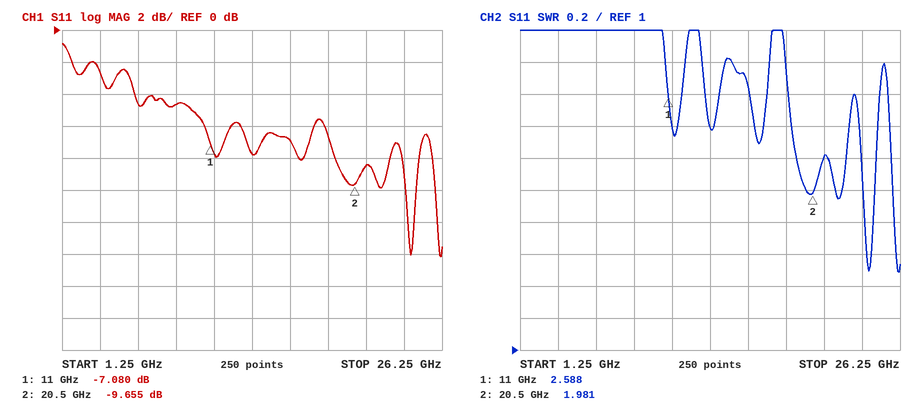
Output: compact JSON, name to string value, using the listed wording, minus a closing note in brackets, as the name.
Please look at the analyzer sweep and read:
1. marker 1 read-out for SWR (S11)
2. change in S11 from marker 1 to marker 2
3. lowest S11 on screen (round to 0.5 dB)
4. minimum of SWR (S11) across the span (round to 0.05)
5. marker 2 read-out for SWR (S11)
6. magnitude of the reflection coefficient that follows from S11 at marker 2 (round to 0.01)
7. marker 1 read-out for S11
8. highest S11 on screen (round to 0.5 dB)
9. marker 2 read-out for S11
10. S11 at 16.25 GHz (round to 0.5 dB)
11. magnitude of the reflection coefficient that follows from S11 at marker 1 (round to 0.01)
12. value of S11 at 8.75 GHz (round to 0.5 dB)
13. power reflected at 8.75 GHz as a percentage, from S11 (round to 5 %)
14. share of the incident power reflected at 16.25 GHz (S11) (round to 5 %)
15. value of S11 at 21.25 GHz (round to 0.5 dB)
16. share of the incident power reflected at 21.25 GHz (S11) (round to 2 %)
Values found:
{"marker 1 read-out for SWR": "2.588", "change in S11 from marker 1 to marker 2": "-2.575 dB", "lowest S11 on screen": "-14.0 dB", "minimum of SWR (S11) across the span": "1.50", "marker 2 read-out for SWR": "1.981", "magnitude of the reflection coefficient that follows from S11 at marker 2": "0.33", "marker 1 read-out for S11": "-7.080 dB", "highest S11 on screen": "-1.0 dB", "marker 2 read-out for S11": "-9.655 dB", "S11 at 16.25 GHz": "-7.0 dB", "magnitude of the reflection coefficient that follows from S11 at marker 1": "0.44", "value of S11 at 8.75 GHz": "-4.5 dB", "power reflected at 8.75 GHz as a percentage, from S11": "35 %", "share of the incident power reflected at 16.25 GHz (S11)": "20 %", "value of S11 at 21.25 GHz": "-8.5 dB", "share of the incident power reflected at 21.25 GHz (S11)": "14 %"}
